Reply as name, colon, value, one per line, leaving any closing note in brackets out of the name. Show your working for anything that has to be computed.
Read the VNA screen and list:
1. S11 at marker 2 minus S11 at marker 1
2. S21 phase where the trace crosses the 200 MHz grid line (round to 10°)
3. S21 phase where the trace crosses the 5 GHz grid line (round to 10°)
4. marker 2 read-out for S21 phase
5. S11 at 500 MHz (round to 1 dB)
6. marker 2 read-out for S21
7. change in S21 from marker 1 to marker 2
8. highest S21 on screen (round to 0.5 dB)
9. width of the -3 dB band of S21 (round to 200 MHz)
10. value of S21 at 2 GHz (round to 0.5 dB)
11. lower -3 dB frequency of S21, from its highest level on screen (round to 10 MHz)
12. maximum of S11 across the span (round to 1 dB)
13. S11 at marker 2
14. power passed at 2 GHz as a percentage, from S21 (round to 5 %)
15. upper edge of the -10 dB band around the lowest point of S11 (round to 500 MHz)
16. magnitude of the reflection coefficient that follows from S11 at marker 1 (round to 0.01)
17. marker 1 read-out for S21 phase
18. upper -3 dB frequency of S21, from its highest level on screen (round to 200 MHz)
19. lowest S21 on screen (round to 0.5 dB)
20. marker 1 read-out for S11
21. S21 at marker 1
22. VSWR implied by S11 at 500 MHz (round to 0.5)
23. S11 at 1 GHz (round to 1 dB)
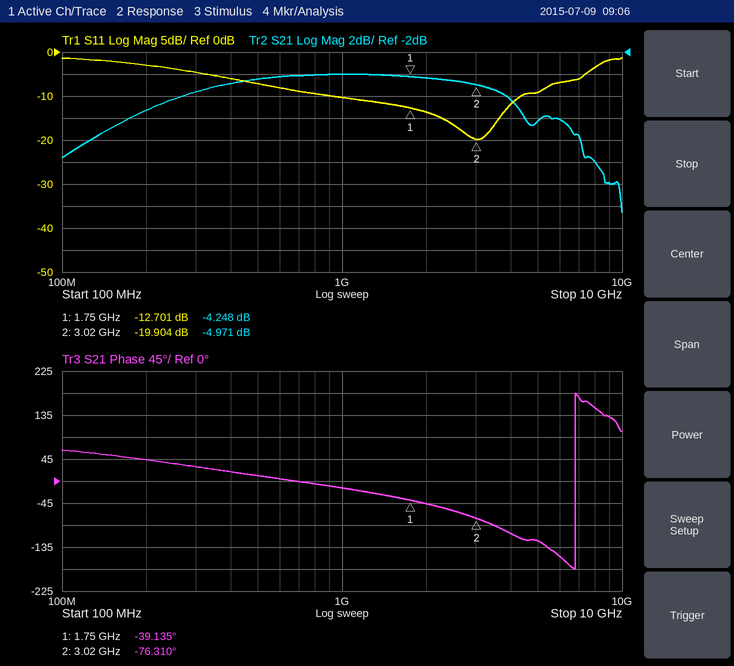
S11 at marker 2 minus S11 at marker 1: -19.904 − (-12.701) = -7.203 dB
S21 phase where the trace crosses the 200 MHz grid line: 40°
S21 phase where the trace crosses the 5 GHz grid line: -120°
marker 2 read-out for S21 phase: -76.310°
S11 at 500 MHz: -7 dB
marker 2 read-out for S21: -4.971 dB
change in S21 from marker 1 to marker 2: -4.971 − (-4.248) = -0.723 dB
highest S21 on screen: -4.0 dB
width of the -3 dB band of S21: 4.2 GHz − 210 MHz = 3.99 GHz
value of S21 at 2 GHz: -4.5 dB
lower -3 dB frequency of S21, from its highest level on screen: 210 MHz
maximum of S11 across the span: -1 dB
S11 at marker 2: -19.904 dB
power passed at 2 GHz as a percentage, from S21: 10^(-4.5/10) ≈ 35 %
upper edge of the -10 dB band around the lowest point of S11: 4.5 GHz
magnitude of the reflection coefficient that follows from S11 at marker 1: 10^(-12.701/20) ≈ 0.23
marker 1 read-out for S21 phase: -39.135°
upper -3 dB frequency of S21, from its highest level on screen: 4.2 GHz
lowest S21 on screen: -16.5 dB
marker 1 read-out for S11: -12.701 dB
S21 at marker 1: -4.248 dB
VSWR implied by S11 at 500 MHz: |Γ| = 10^(-7/20) = 0.4467; VSWR = (1 + 0.4467)/(1 − 0.4467) ≈ 2.61, so 2.5 to the nearest 0.5
S11 at 1 GHz: -10 dB
